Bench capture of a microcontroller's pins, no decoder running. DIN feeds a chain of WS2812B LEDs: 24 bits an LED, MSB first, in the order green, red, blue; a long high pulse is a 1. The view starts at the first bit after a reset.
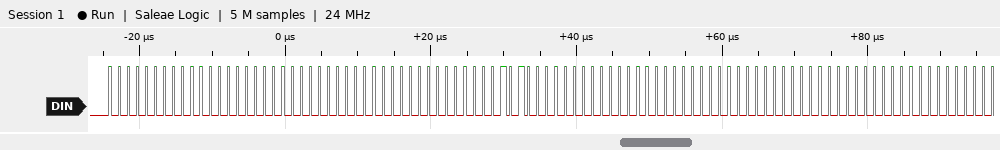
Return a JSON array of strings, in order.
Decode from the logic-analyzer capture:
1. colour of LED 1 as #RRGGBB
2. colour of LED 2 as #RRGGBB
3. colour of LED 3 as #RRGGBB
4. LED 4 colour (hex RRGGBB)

["#000000", "#000014", "#000000", "#000000"]
